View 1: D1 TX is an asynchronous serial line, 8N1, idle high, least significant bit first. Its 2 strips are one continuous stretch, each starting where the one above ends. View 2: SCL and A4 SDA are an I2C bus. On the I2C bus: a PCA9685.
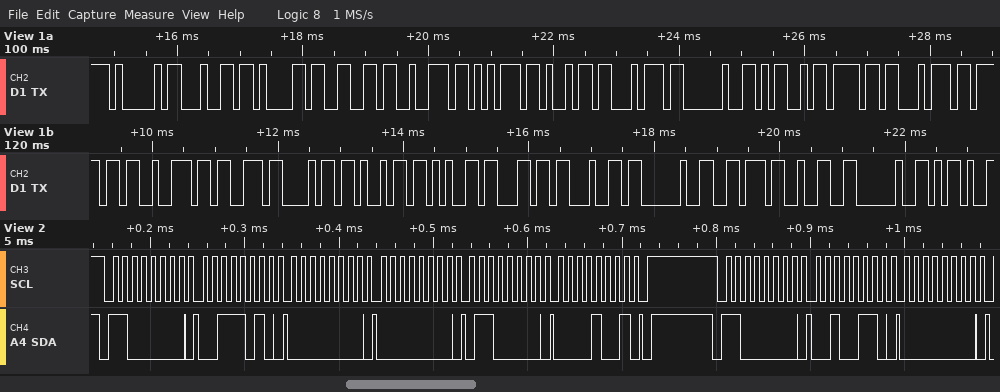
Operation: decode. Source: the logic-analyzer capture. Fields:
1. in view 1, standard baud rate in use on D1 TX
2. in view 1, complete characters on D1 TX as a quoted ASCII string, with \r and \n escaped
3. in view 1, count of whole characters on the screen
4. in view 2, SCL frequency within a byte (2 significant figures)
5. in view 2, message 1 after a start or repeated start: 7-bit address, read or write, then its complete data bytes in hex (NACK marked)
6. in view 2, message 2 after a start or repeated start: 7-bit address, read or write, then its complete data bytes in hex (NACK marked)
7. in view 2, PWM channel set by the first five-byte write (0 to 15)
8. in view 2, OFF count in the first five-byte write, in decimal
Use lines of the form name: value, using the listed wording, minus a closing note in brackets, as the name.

in view 1, standard baud rate in use on D1 TX: 9600 baud
in view 1, complete characters on D1 TX as a quoted ASCII string, with \r and \n escaped: "Adafruit Motorshield v2 -"
in view 1, count of whole characters on the screen: 25
in view 2, SCL frequency within a byte: 100 kHz
in view 2, message 1 after a start or repeated start: 7-bit address, read or write, then its complete data bytes in hex: 0x60 write: 3A 00 00 60 09
in view 2, message 2 after a start or repeated start: 7-bit address, read or write, then its complete data bytes in hex: 0x60 write: 26 00
in view 2, PWM channel set by the first five-byte write: 13
in view 2, OFF count in the first five-byte write, in decimal: 2400
